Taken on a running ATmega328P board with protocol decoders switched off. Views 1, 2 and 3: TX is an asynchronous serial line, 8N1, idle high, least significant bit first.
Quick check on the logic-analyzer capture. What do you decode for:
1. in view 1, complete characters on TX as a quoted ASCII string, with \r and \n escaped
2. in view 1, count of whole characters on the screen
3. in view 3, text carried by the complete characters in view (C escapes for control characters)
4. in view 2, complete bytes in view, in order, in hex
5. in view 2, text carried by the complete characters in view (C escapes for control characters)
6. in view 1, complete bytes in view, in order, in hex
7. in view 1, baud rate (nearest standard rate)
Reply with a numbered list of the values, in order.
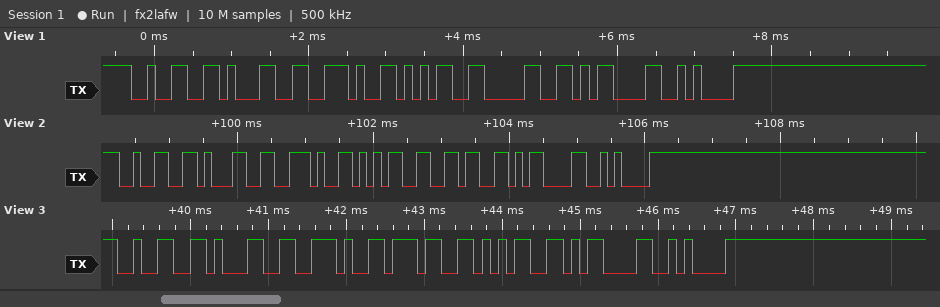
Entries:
1. "21.50\r\n"
2. 7
3. "21.75\r\n"
4. 0x32 0x31 0x2E 0x35 0x36 0x0D 0x0A
5. "21.56\r\n"
6. 32 31 2E 35 30 0D 0A
7. 9600 baud
